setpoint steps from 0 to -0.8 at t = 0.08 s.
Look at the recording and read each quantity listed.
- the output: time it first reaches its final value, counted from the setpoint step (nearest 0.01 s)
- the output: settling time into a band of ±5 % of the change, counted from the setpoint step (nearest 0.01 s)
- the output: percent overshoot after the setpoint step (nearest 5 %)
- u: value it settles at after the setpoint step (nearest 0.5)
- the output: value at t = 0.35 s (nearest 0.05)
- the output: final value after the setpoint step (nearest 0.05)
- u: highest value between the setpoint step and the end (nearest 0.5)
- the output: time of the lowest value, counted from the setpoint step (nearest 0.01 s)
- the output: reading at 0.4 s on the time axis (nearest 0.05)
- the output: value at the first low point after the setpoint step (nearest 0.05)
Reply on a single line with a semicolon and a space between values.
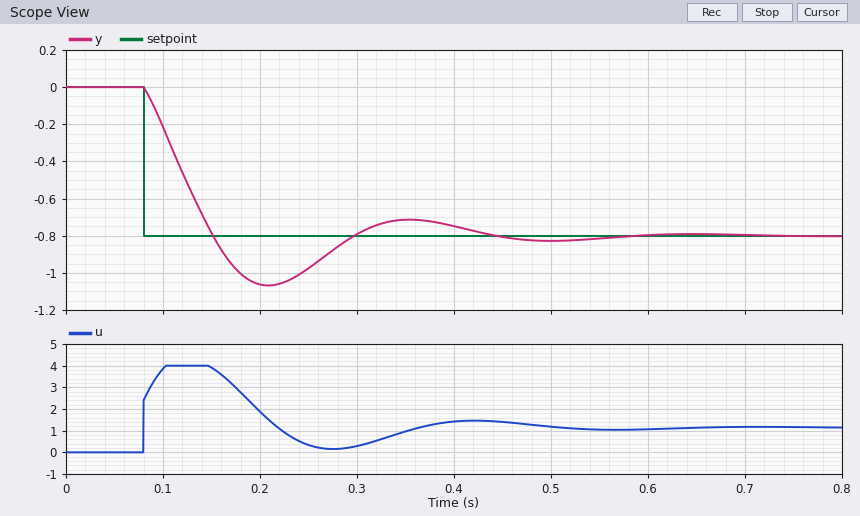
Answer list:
0.07 s; 0.33 s; 35 %; 1.0; -0.70; -0.80; 4.0; 0.13 s; -0.75; -1.05
